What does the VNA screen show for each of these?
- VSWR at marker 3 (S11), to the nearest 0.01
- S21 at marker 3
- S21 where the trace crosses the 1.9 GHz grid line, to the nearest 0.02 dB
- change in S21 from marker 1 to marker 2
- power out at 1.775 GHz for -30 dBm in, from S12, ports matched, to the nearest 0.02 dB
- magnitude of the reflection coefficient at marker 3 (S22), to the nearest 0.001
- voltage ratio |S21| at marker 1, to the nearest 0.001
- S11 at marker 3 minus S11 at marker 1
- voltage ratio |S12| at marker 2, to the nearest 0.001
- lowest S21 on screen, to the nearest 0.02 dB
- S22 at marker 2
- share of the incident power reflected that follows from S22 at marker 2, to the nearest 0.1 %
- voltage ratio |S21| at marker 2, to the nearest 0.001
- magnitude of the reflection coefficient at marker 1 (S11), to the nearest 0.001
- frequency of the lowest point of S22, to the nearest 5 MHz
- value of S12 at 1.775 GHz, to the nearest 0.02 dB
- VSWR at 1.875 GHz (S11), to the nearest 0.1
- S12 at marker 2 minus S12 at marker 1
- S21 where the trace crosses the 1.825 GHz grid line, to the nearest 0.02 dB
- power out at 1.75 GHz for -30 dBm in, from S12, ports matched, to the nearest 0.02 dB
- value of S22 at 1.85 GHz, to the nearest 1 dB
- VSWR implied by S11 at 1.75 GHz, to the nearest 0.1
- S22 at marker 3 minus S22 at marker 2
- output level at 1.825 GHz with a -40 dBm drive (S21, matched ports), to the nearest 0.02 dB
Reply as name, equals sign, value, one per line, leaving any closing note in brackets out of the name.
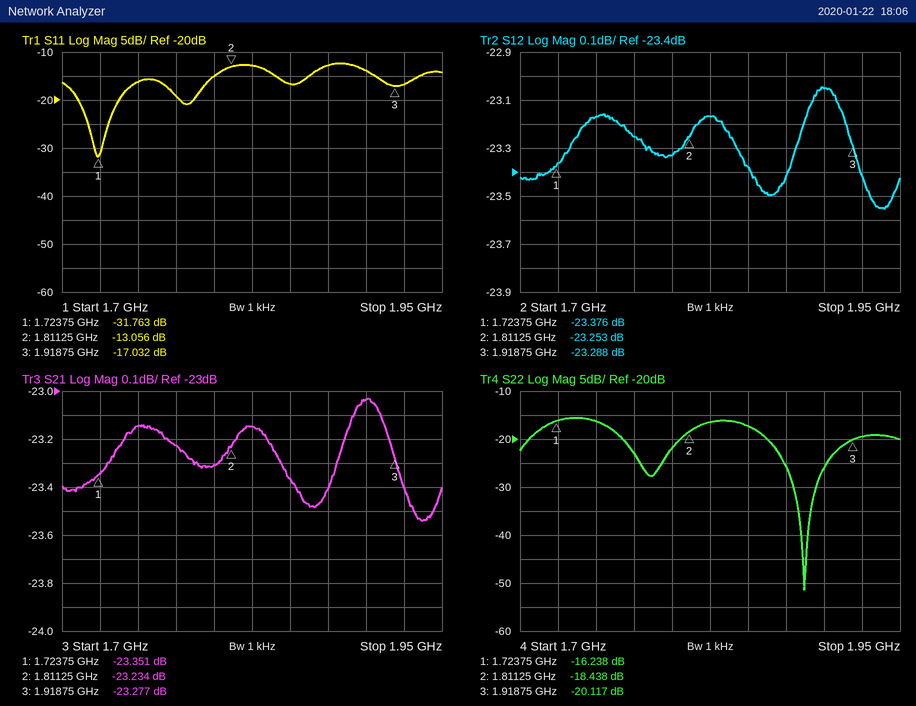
VSWR at marker 3 (S11), to the nearest 0.01 = 1.33
S21 at marker 3 = -23.277 dB
S21 where the trace crosses the 1.9 GHz grid line, to the nearest 0.02 dB = -23.04 dB
change in S21 from marker 1 to marker 2 = 0.117 dB
power out at 1.775 GHz for -30 dBm in, from S12, ports matched, to the nearest 0.02 dB = -53.26 dBm
magnitude of the reflection coefficient at marker 3 (S22), to the nearest 0.001 = 0.099
voltage ratio |S21| at marker 1, to the nearest 0.001 = 0.068
S11 at marker 3 minus S11 at marker 1 = 14.731 dB
voltage ratio |S12| at marker 2, to the nearest 0.001 = 0.069
lowest S21 on screen, to the nearest 0.02 dB = -23.54 dB
S22 at marker 2 = -18.438 dB
share of the incident power reflected that follows from S22 at marker 2, to the nearest 0.1 % = 1.4 %
voltage ratio |S21| at marker 2, to the nearest 0.001 = 0.069
magnitude of the reflection coefficient at marker 1 (S11), to the nearest 0.001 = 0.026
frequency of the lowest point of S22, to the nearest 5 MHz = 1.885 GHz
value of S12 at 1.775 GHz, to the nearest 0.02 dB = -23.26 dB
VSWR at 1.875 GHz (S11), to the nearest 0.1 = 1.6
S12 at marker 2 minus S12 at marker 1 = 0.123 dB
S21 where the trace crosses the 1.825 GHz grid line, to the nearest 0.02 dB = -23.14 dB
power out at 1.75 GHz for -30 dBm in, from S12, ports matched, to the nearest 0.02 dB = -53.16 dBm
value of S22 at 1.85 GHz, to the nearest 1 dB = -17 dB
VSWR implied by S11 at 1.75 GHz, to the nearest 0.1 = 1.4
S22 at marker 3 minus S22 at marker 2 = -1.679 dB
output level at 1.825 GHz with a -40 dBm drive (S21, matched ports), to the nearest 0.02 dB = -63.14 dBm
